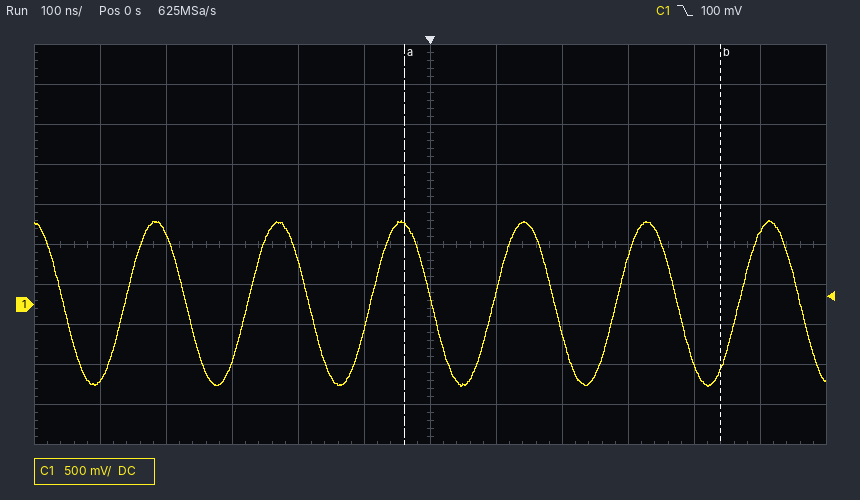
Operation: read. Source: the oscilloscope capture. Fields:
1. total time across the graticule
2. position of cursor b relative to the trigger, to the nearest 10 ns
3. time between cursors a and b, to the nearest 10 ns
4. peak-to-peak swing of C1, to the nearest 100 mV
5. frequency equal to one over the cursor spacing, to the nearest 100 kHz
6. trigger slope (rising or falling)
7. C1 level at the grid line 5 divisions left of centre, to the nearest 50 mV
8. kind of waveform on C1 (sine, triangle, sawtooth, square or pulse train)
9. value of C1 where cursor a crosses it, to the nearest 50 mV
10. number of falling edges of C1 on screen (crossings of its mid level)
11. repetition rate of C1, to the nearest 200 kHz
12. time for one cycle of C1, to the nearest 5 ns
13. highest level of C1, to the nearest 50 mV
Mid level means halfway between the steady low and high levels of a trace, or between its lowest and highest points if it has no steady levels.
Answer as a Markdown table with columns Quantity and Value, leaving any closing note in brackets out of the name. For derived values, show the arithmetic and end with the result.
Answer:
| Quantity | Value |
|---|---|
| total time across the graticule | 1.2 µs |
| position of cursor b relative to the trigger, to the nearest 10 ns | +440 ns |
| time between cursors a and b, to the nearest 10 ns | 480 ns |
| peak-to-peak swing of C1, to the nearest 100 mV | 2.10 V |
| frequency equal to one over the cursor spacing, to the nearest 100 kHz | 1 / 480 ns ≈ 2.1 MHz |
| trigger slope | falling |
| C1 level at the grid line 5 divisions left of centre, to the nearest 50 mV | -950 mV |
| kind of waveform on C1 | sine |
| value of C1 where cursor a crosses it, to the nearest 50 mV | 1.00 V |
| number of falling edges of C1 on screen | 7 |
| repetition rate of C1, to the nearest 200 kHz | 1 / 185 ns ≈ 5.4 MHz |
| time for one cycle of C1, to the nearest 5 ns | 185 ns |
| highest level of C1, to the nearest 50 mV | 1.05 V |
